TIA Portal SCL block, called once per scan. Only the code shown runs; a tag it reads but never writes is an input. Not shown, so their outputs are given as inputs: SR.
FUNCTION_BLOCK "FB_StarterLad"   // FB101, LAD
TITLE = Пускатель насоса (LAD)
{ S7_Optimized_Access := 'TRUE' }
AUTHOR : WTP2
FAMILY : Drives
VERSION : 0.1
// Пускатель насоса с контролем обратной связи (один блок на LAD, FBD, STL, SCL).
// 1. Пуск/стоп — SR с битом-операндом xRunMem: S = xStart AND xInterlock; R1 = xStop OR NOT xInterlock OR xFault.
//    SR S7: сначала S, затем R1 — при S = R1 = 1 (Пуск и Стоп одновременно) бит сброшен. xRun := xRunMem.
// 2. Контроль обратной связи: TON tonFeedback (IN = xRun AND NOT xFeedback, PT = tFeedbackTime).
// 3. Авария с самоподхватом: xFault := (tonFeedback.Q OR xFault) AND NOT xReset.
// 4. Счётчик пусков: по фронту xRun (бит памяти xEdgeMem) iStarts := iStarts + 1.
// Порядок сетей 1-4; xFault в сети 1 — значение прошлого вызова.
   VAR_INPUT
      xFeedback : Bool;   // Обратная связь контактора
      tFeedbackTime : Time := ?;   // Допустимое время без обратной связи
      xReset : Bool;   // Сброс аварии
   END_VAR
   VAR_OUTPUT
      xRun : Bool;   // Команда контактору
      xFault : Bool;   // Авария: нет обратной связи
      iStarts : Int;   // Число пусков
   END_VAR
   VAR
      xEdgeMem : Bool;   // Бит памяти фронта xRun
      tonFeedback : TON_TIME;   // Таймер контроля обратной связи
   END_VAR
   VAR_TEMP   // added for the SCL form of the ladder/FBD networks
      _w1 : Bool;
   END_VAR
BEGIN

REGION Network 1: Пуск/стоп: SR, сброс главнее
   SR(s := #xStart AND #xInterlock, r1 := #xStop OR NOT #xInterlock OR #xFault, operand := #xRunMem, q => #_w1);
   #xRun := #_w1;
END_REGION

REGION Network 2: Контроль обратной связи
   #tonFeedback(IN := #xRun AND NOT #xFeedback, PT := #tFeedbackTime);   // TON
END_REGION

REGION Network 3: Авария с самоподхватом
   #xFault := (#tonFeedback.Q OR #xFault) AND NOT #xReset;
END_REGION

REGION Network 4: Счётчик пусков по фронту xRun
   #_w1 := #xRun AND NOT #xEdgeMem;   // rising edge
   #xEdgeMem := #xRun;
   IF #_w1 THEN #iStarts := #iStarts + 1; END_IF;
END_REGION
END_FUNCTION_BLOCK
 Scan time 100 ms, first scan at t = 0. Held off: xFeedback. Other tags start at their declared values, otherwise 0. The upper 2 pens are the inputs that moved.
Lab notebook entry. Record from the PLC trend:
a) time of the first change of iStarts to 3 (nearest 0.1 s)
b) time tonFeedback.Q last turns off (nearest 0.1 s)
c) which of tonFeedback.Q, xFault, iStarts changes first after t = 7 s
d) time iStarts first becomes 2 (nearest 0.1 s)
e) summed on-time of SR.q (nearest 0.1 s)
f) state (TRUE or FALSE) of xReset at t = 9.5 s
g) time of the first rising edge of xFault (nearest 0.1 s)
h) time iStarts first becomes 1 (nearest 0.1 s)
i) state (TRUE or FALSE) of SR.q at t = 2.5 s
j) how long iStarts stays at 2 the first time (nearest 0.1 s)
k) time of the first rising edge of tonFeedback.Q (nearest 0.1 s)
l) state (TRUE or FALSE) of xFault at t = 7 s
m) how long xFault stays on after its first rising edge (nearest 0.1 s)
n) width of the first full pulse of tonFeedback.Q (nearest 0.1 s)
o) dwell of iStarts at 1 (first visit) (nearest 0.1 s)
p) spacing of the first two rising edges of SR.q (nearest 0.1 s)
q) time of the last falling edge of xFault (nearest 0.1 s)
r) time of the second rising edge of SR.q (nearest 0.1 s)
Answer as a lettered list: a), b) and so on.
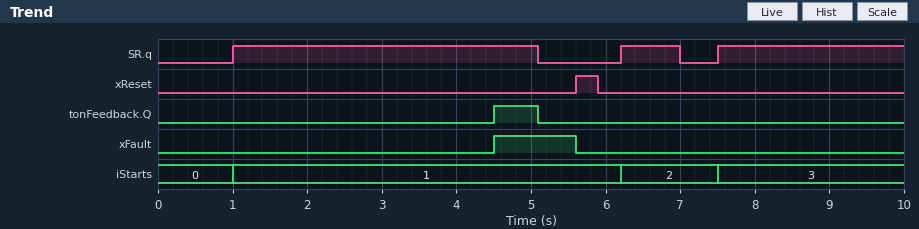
a) 7.5 s
b) 5.1 s
c) iStarts
d) 6.2 s
e) 7.4 s
f) FALSE
g) 4.5 s
h) 1.0 s
i) TRUE
j) 1.3 s
k) 4.5 s
l) FALSE
m) 1.1 s
n) 0.6 s
o) 5.2 s
p) 5.2 s
q) 5.6 s
r) 6.2 s
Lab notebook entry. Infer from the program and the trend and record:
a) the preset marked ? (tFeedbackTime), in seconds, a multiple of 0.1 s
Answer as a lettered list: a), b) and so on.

a) 3.5 s
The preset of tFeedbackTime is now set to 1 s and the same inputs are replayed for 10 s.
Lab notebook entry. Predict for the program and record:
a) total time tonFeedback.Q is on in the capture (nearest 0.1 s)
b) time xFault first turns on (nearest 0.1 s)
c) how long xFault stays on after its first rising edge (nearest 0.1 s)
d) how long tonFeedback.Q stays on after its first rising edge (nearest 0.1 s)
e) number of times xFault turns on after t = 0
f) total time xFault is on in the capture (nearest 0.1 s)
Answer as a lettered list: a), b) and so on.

a) 4.6 s
b) 2.0 s
c) 3.6 s
d) 3.1 s
e) 2
f) 5.1 s
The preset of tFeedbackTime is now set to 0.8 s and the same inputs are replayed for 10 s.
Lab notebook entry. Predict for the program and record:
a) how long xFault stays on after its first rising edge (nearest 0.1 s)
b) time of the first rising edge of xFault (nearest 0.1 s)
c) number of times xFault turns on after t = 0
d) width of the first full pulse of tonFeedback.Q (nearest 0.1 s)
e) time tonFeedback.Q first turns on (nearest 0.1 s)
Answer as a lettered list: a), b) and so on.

a) 3.8 s
b) 1.8 s
c) 2
d) 3.3 s
e) 1.8 s
